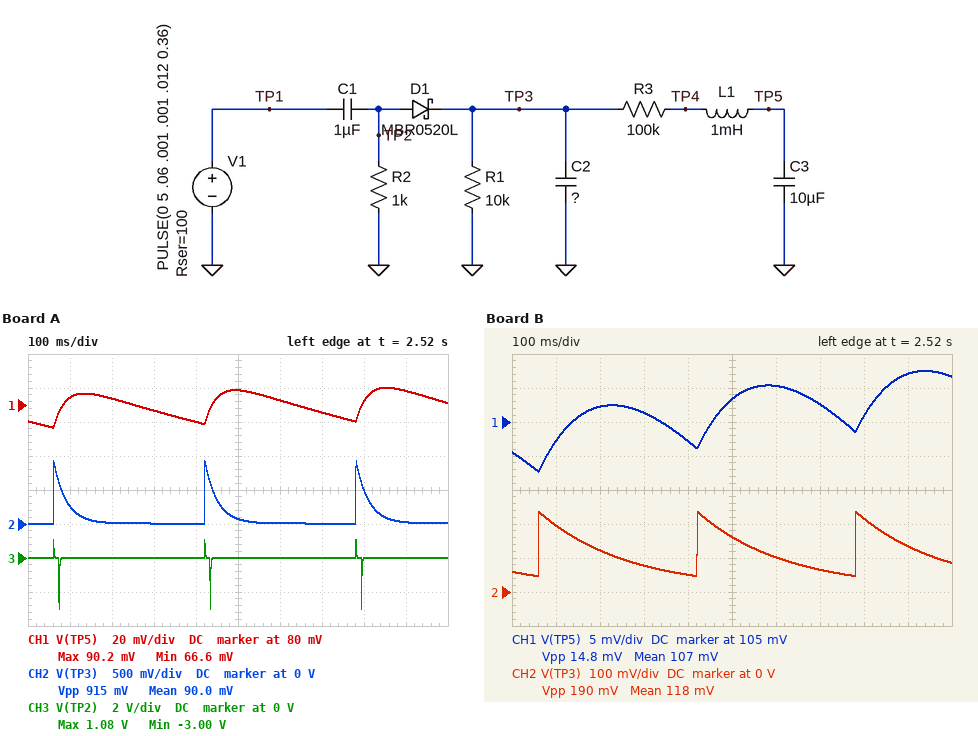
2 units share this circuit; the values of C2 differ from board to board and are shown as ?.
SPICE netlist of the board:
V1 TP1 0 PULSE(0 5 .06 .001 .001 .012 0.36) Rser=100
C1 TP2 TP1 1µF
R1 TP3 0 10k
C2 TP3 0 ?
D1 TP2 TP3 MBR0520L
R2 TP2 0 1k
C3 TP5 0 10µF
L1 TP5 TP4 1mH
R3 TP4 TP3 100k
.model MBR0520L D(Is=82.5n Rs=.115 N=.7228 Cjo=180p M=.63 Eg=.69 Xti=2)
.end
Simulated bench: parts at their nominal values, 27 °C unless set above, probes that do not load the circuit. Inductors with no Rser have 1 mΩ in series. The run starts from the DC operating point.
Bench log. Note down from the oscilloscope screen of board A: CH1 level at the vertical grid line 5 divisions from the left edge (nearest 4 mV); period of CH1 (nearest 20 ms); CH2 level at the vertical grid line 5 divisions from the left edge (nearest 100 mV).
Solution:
88 mV
360 ms
100 mV
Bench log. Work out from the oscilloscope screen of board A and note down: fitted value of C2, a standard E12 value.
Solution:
3.3 µF
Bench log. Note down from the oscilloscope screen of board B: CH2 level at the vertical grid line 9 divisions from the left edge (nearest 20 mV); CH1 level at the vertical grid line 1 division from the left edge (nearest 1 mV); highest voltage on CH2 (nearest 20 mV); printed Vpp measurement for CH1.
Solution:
140 mV
102 mV
240 mV
14.8 mV
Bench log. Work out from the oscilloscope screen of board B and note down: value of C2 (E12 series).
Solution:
22 µF
